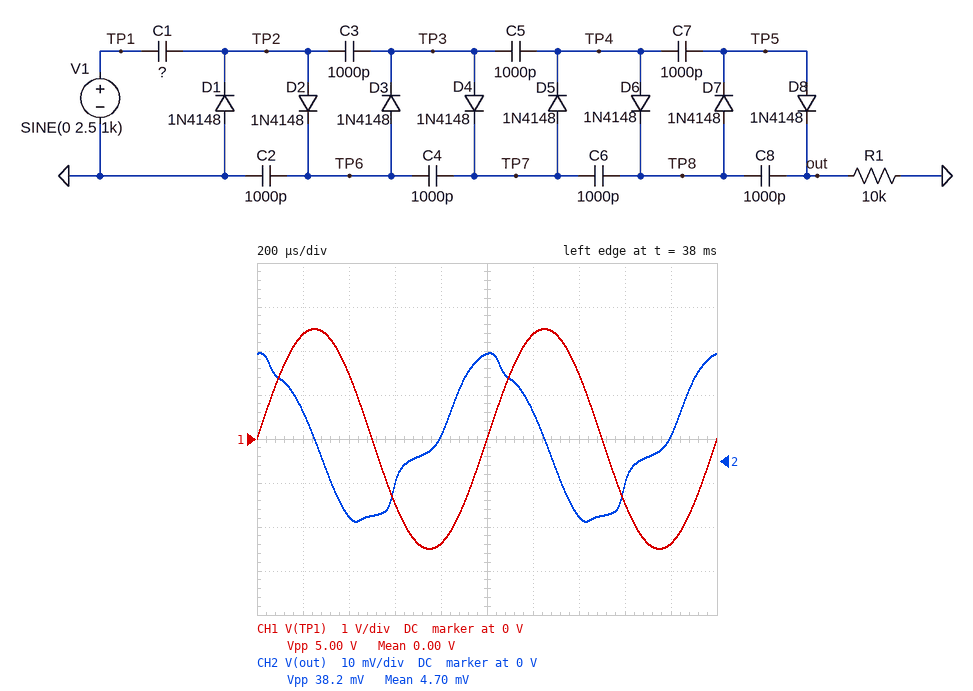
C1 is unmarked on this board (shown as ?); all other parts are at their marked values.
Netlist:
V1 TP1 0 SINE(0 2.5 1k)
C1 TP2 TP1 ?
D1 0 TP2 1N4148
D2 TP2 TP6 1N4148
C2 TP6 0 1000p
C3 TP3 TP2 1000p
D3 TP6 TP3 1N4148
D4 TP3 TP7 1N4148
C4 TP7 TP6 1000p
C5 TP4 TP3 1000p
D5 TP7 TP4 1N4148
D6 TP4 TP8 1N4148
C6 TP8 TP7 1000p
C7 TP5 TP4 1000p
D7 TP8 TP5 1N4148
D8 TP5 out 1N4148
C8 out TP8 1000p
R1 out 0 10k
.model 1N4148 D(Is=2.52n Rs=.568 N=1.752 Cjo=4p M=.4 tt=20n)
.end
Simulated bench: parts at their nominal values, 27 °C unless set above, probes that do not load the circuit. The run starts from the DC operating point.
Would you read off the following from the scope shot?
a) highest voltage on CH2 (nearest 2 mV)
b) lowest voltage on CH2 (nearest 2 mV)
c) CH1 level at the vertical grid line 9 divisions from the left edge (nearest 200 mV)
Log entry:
24 mV
-14 mV
-2.4 V
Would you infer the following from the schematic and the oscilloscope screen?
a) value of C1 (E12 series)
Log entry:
390 pF
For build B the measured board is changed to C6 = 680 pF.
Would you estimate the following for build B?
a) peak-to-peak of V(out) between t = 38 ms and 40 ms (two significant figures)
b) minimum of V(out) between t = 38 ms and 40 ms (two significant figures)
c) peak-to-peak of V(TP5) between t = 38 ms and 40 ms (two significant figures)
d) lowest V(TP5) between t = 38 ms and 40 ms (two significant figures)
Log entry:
37 mV
-13 mV
350 mV
-44 mV
